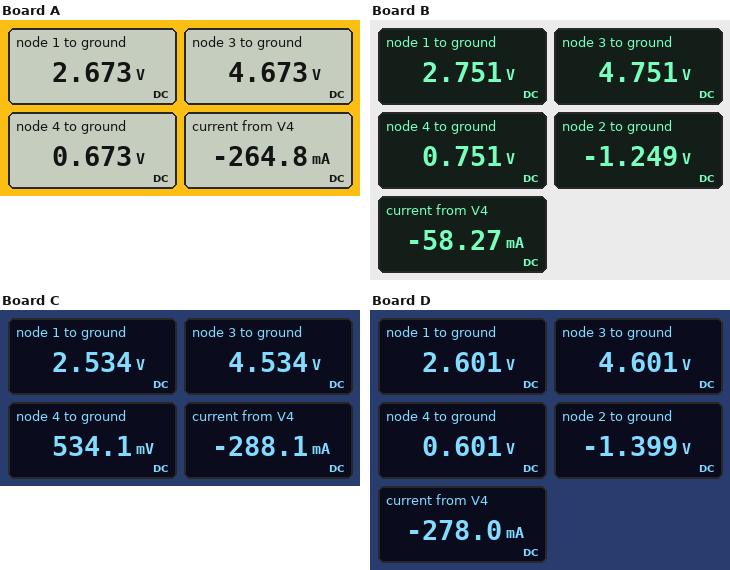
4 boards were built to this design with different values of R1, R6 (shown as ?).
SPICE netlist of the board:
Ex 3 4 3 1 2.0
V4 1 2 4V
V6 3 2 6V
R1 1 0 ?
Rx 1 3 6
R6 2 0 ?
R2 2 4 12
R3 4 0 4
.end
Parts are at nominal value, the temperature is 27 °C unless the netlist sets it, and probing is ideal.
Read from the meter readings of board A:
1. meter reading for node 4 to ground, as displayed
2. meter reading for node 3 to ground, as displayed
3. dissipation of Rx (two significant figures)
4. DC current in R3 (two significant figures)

0.673 V
4.673 V
670 mW
170 mA
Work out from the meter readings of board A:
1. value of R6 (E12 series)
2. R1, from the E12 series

5.6 Ω
39 Ω
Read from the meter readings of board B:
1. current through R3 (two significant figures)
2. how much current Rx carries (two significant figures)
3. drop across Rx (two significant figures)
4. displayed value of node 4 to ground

190 mA
330 mA
2.0 V
0.751 V
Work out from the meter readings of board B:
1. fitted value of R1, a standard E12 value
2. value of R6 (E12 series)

10 Ω
2.7 Ω
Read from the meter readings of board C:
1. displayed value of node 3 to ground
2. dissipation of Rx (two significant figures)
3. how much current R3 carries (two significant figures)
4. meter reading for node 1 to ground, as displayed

4.534 V
670 mW
130 mA
2.534 V
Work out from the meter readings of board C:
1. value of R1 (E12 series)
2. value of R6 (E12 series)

56 Ω
8.2 Ω
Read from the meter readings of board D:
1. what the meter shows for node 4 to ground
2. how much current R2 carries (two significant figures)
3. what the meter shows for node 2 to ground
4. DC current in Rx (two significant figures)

0.601 V
170 mA
-1.399 V
330 mA
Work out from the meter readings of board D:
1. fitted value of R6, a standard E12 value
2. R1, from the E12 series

6.8 Ω
47 Ω
